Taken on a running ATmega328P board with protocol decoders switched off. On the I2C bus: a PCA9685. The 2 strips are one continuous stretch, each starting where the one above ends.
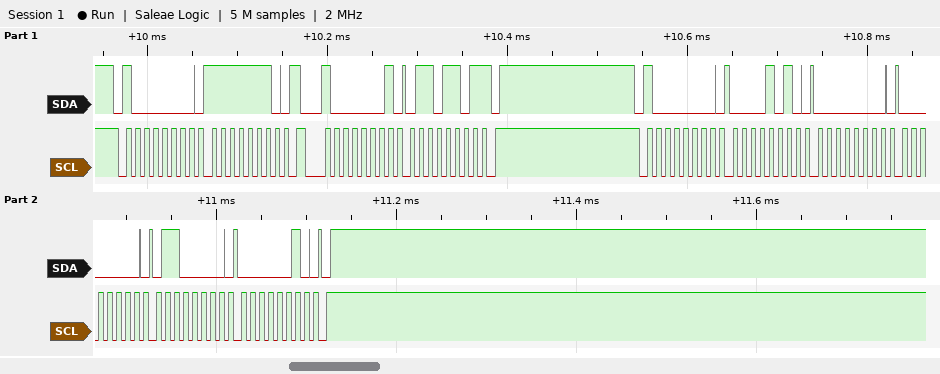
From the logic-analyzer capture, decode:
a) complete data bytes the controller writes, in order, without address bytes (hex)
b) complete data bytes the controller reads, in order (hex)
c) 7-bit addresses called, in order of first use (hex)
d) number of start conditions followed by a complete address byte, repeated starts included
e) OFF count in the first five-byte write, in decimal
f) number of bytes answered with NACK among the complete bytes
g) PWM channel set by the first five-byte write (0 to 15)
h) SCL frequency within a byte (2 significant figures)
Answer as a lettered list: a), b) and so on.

a) FE 0A 00 00 60 02
b) 6D
c) 0x40
d) 3
e) 608
f) 1
g) 1
h) 100 kHz
